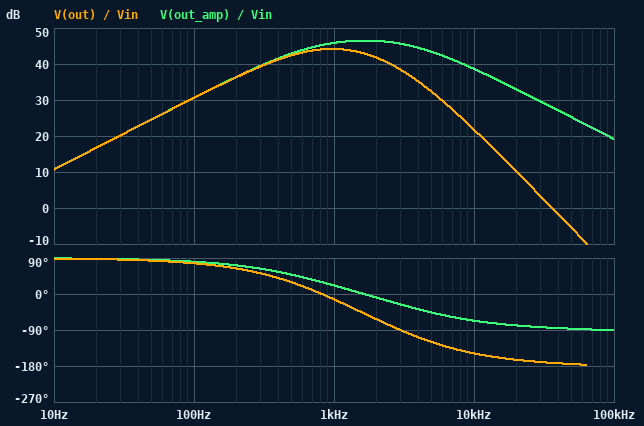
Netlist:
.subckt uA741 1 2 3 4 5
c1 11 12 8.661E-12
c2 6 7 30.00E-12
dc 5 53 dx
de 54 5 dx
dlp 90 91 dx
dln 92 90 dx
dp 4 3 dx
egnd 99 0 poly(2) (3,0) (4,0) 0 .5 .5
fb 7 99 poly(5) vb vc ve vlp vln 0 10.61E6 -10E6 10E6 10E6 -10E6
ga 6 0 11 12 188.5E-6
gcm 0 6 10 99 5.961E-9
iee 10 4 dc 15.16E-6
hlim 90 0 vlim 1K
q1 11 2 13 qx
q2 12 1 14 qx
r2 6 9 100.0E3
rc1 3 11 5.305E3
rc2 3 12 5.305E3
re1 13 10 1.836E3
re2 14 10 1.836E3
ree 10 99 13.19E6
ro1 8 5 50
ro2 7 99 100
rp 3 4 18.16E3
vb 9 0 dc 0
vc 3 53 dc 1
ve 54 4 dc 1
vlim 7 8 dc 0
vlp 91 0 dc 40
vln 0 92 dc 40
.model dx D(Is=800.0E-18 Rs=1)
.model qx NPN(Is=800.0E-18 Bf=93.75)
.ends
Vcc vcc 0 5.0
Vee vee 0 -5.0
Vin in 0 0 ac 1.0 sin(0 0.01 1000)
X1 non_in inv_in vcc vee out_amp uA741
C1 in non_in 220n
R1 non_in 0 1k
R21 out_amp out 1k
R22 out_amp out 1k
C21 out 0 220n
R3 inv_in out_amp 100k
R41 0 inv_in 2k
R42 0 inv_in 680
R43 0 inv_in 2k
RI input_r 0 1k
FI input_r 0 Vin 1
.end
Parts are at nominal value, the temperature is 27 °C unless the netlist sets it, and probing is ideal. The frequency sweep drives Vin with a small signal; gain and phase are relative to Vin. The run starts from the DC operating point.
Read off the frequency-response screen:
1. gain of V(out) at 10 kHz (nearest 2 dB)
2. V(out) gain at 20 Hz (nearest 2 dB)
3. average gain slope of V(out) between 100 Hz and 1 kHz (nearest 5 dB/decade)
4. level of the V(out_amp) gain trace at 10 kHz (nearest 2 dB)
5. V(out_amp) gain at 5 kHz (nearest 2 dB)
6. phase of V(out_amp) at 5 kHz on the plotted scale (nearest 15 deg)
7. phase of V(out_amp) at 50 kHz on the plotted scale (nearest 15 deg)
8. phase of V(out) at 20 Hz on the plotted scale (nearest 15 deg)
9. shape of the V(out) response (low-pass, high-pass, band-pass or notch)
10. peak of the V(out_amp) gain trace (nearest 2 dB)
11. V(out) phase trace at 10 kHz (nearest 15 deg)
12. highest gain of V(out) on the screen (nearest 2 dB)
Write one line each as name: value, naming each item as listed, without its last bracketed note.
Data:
gain of V(out) at 10 kHz: 22 dB
V(out) gain at 20 Hz: 16 dB
average gain slope of V(out) between 100 Hz and 1 kHz: 15 dB/decade
level of the V(out_amp) gain trace at 10 kHz: 38 dB
V(out_amp) gain at 5 kHz: 44 dB
phase of V(out_amp) at 5 kHz on the plotted scale: -45 deg
phase of V(out_amp) at 50 kHz on the plotted scale: -90 deg
phase of V(out) at 20 Hz on the plotted scale: 90 deg
shape of the V(out) response: band-pass
peak of the V(out_amp) gain trace: 46 dB
V(out) phase trace at 10 kHz: -150 deg
highest gain of V(out) on the screen: 44 dB
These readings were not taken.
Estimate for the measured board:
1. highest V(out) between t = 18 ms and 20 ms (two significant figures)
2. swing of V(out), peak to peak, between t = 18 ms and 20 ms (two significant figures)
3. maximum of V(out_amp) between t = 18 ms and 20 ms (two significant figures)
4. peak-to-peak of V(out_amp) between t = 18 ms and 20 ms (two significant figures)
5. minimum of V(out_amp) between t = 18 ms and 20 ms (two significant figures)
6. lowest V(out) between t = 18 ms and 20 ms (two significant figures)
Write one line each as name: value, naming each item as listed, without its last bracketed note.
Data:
highest V(out) between t = 18 ms and 20 ms: 1.6 V
swing of V(out), peak to peak, between t = 18 ms and 20 ms: 3.2 V
maximum of V(out_amp) between t = 18 ms and 20 ms: 2.0 V
peak-to-peak of V(out_amp) between t = 18 ms and 20 ms: 3.9 V
minimum of V(out_amp) between t = 18 ms and 20 ms: -2.0 V
lowest V(out) between t = 18 ms and 20 ms: -1.6 V
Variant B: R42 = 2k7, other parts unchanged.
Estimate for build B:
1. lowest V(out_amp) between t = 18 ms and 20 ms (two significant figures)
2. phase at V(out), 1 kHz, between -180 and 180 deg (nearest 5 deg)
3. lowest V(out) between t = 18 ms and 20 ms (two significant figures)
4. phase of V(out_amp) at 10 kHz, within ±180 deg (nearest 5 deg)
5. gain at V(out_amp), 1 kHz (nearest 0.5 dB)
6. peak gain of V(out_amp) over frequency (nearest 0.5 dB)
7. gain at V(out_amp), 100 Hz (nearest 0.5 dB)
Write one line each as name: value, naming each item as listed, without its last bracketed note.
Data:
lowest V(out_amp) between t = 18 ms and 20 ms: -1.1 V
phase at V(out), 1 kHz, between -180 and 180 deg: -5 deg
lowest V(out) between t = 18 ms and 20 ms: -920 mV
phase of V(out_amp) at 10 kHz, within ±180 deg: -55 deg
gain at V(out_amp), 1 kHz: 41.0 dB
peak gain of V(out_amp) over frequency: 42.0 dB
gain at V(out_amp), 100 Hz: 25.5 dB
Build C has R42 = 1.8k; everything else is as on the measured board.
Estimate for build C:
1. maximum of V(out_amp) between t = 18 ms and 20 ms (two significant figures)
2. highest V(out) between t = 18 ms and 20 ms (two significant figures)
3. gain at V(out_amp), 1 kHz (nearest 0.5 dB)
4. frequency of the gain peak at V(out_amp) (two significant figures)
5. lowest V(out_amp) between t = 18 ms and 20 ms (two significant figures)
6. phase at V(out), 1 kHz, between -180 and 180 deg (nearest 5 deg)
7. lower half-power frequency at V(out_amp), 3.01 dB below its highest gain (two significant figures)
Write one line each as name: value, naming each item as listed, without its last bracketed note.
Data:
maximum of V(out_amp) between t = 18 ms and 20 ms: 1.3 V
highest V(out) between t = 18 ms and 20 ms: 1.0 V
gain at V(out_amp), 1 kHz: 42.0 dB
frequency of the gain peak at V(out_amp): 2.1 kHz
lowest V(out_amp) between t = 18 ms and 20 ms: -1.3 V
phase at V(out), 1 kHz, between -180 and 180 deg: -10 deg
lower half-power frequency at V(out_amp), 3.01 dB below its highest gain: 600 Hz
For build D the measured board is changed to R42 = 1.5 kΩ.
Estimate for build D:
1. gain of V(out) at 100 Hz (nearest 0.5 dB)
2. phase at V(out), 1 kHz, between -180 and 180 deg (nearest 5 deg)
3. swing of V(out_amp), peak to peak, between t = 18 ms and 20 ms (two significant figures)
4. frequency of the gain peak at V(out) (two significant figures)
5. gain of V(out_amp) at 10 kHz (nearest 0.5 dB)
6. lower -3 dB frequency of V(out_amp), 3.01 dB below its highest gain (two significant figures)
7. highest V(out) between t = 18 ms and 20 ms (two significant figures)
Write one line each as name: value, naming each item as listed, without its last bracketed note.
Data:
gain of V(out) at 100 Hz: 27.0 dB
phase at V(out), 1 kHz, between -180 and 180 deg: -10 deg
swing of V(out_amp), peak to peak, between t = 18 ms and 20 ms: 2.7 V
frequency of the gain peak at V(out): 1.0 kHz
gain of V(out_amp) at 10 kHz: 38.0 dB
lower -3 dB frequency of V(out_amp), 3.01 dB below its highest gain: 600 Hz
highest V(out) between t = 18 ms and 20 ms: 1.1 V
